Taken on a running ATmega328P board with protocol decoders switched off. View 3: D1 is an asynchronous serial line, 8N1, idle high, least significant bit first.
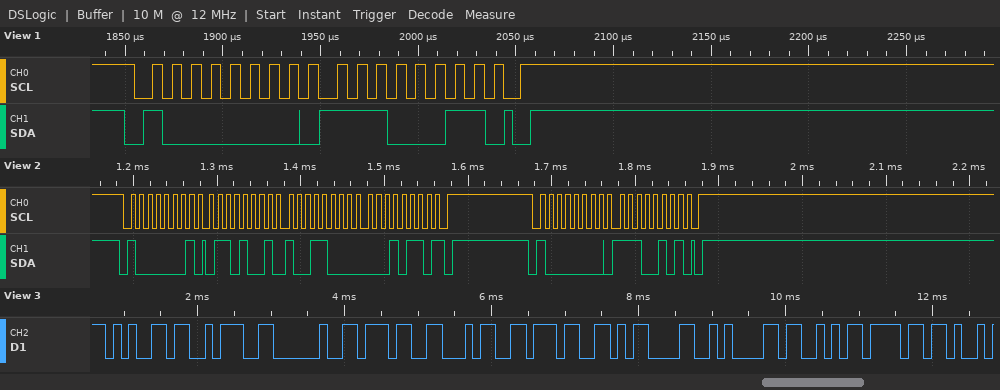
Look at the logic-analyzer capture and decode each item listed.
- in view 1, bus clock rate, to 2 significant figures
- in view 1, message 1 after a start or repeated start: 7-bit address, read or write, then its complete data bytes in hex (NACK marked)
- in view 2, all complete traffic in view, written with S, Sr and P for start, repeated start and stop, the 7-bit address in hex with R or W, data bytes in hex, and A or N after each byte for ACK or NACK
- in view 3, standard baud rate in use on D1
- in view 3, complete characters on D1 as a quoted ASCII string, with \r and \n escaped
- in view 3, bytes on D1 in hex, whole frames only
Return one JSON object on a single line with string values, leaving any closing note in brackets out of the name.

{"in view 1, bus clock rate, to 2 significant figures": "100 kHz", "in view 1, message 1 after a start or repeated start: 7-bit address, read or write, then its complete data bytes in hex": "0x40 write: E3", "in view 2, all complete traffic in view, written with S, Sr and P for start, repeated start and stop, the 7-bit address in hex with R or W, data bytes in hex, and A or N after each byte for ACK or NACK": "S 40R A 69 A 98 A 16 N P S 40W A E5 A P", "in view 3, standard baud rate in use on D1": "9600 baud", "in view 3, complete characters on D1 as a quoted ASCII string, with \\r and \\n escaped": "\"e: 747\\r\\nSo\"", "in view 3, bytes on D1 in hex, whole frames only": "65 3A 20 37 34 37 0D 0A 53 6F"}
